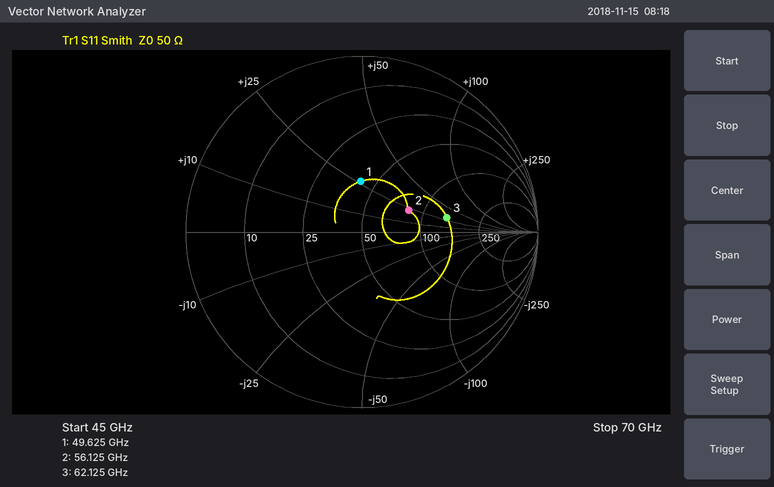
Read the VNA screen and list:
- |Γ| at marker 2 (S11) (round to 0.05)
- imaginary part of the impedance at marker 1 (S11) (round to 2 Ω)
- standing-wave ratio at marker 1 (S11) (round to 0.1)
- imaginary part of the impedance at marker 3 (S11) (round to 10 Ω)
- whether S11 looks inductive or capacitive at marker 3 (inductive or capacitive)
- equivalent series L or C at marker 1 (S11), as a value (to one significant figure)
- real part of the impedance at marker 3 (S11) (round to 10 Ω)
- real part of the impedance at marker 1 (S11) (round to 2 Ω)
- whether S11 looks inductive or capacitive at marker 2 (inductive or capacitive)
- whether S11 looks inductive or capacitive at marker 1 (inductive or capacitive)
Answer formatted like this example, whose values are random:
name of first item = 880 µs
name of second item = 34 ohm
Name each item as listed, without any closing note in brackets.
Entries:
|Γ| at marker 2 (S11) = 0.30
imaginary part of the impedance at marker 1 (S11) = +26 Ω
standing-wave ratio at marker 1 (S11) = 1.8
imaginary part of the impedance at marker 3 (S11) = +30 Ω
whether S11 looks inductive or capacitive at marker 3 = inductive
equivalent series L or C at marker 1 (S11), as a value = 80 pH
real part of the impedance at marker 3 (S11) = 140 Ω
real part of the impedance at marker 1 (S11) = 42 Ω
whether S11 looks inductive or capacitive at marker 2 = inductive
whether S11 looks inductive or capacitive at marker 1 = inductive
